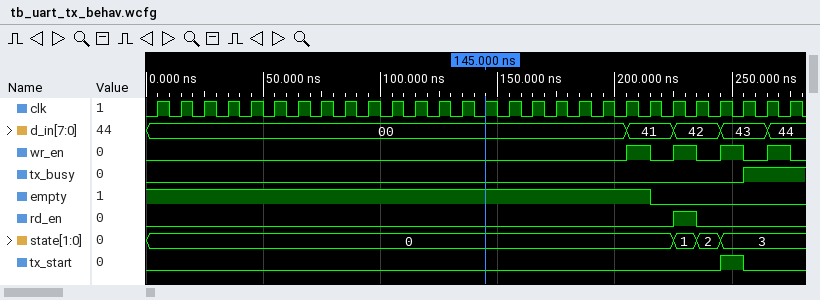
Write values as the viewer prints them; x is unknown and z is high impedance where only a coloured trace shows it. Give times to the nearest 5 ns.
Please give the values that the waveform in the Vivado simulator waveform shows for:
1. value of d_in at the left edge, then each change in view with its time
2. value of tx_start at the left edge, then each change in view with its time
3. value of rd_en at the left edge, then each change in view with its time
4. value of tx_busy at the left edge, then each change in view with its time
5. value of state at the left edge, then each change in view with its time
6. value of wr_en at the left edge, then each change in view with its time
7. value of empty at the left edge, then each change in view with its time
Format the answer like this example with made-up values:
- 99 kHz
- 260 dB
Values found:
- 00, 41 at 205 ns, 42 at 225 ns, 43 at 245 ns, 44 at 265 ns
- 0, 1 at 245 ns, 0 at 255 ns
- 0, 1 at 225 ns, 0 at 235 ns
- 0, 1 at 255 ns
- 0, 1 at 225 ns, 2 at 235 ns, 3 at 245 ns
- 0, 1 at 205 ns, 0 at 215 ns, 1 at 225 ns, 0 at 235 ns, 1 at 245 ns, 0 at 255 ns, 1 at 265 ns, 0 at 275 ns
- 1, 0 at 215 ns
